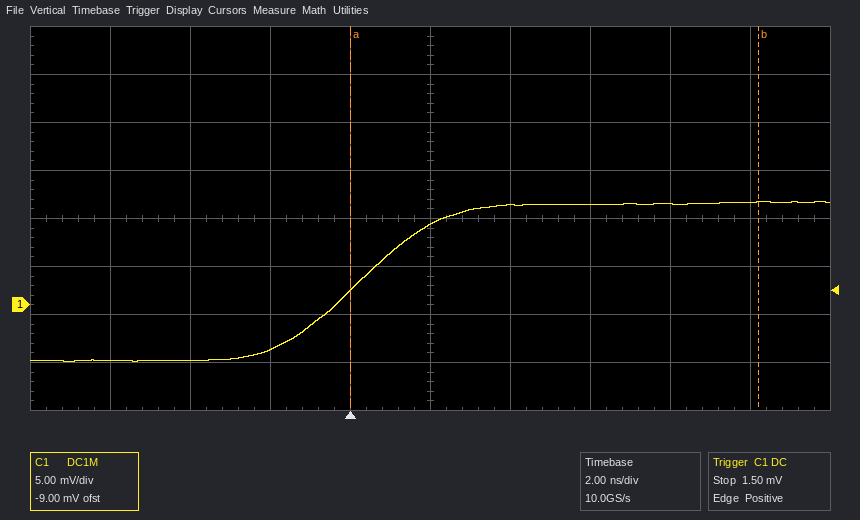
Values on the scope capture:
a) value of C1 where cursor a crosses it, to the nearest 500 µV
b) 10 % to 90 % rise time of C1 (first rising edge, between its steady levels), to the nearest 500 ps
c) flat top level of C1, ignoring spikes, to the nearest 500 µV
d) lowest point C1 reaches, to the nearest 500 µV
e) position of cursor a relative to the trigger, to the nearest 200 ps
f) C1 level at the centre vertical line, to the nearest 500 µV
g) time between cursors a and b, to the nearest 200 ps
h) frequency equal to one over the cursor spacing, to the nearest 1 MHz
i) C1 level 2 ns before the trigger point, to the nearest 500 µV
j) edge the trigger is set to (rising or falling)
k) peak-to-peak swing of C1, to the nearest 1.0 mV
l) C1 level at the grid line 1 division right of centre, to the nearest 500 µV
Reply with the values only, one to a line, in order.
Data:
1.5 mV
4.0 ns
10.5 mV
-6.0 mV
0.0 ns
8.5 mV
10.2 ns
98 MHz
-4.5 mV
rising
17.0 mV
10.5 mV
